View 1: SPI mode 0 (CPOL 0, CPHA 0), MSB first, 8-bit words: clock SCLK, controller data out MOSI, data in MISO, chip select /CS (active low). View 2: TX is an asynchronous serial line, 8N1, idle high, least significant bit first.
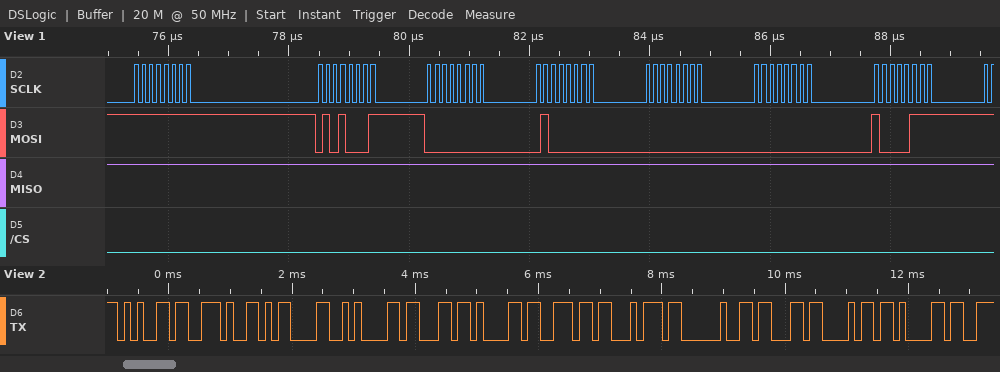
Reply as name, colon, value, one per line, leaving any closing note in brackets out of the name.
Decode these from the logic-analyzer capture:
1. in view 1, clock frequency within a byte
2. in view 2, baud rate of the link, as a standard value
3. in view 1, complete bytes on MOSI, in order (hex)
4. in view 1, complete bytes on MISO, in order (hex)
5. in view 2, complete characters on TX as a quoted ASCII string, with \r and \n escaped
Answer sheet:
in view 1, clock frequency within a byte: 8 MHz
in view 2, baud rate of the link, as a standard value: 9600 baud
in view 1, complete bytes on MOSI, in order: FF 51 00 40 00 00 87
in view 1, complete bytes on MISO, in order: FF FF FF FF FF FF FF
in view 2, complete characters on TX as a quoted ASCII string, with \r and \n escaped: "e.\r\ncant cha"
